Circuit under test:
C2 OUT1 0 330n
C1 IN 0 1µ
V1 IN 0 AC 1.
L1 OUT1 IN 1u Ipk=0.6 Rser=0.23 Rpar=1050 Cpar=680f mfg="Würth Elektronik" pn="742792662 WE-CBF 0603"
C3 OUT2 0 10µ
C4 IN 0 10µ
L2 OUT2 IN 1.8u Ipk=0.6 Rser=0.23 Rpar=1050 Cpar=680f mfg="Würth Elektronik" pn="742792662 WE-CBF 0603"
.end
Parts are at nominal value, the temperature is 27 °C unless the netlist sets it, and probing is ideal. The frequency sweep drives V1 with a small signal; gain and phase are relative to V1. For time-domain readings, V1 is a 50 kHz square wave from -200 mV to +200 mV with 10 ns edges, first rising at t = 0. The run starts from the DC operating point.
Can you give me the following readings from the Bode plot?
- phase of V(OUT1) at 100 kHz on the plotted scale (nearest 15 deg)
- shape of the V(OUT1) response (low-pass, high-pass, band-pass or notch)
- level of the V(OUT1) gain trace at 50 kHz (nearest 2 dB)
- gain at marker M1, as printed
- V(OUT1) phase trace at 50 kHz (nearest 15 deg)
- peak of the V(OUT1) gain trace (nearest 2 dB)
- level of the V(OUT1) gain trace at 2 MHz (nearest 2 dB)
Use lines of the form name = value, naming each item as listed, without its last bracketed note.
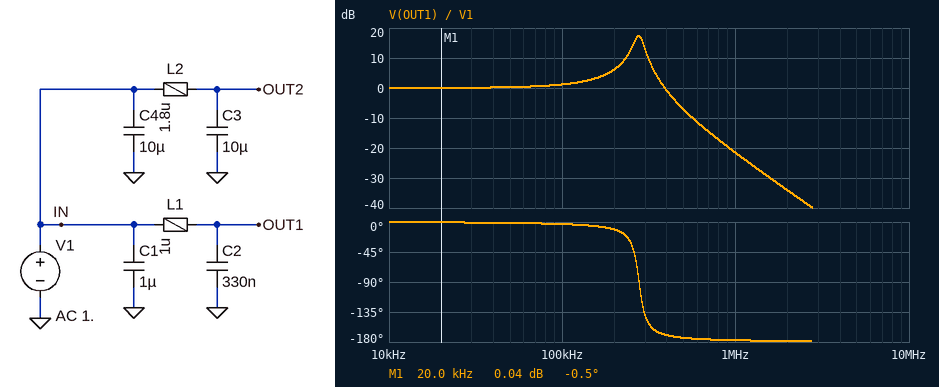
phase of V(OUT1) at 100 kHz on the plotted scale = 0 deg
shape of the V(OUT1) response = low-pass
level of the V(OUT1) gain trace at 50 kHz = 0 dB
gain at marker M1, as printed = 0.04 dB
V(OUT1) phase trace at 50 kHz = 0 deg
peak of the V(OUT1) gain trace = 18 dB
level of the V(OUT1) gain trace at 2 MHz = -34 dB
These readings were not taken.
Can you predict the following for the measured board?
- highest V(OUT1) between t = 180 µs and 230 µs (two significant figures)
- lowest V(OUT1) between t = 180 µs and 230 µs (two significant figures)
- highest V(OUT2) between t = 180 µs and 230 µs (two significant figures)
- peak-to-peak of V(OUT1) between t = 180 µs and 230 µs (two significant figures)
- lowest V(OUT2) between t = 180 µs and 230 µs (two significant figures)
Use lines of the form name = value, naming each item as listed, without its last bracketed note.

highest V(OUT1) between t = 180 µs and 230 µs = 510 mV
lowest V(OUT1) between t = 180 µs and 230 µs = -510 mV
highest V(OUT2) between t = 180 µs and 230 µs = 240 mV
peak-to-peak of V(OUT1) between t = 180 µs and 230 µs = 1.0 V
lowest V(OUT2) between t = 180 µs and 230 µs = -240 mV
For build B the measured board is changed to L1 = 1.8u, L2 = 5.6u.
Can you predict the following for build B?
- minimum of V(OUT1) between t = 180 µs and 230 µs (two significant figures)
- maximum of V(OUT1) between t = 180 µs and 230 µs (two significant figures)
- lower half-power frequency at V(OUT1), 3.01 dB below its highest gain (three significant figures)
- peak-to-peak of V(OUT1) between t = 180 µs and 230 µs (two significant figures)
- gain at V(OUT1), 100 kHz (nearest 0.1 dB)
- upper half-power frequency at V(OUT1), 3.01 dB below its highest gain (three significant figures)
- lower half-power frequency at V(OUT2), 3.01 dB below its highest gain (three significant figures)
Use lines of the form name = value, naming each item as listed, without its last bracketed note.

minimum of V(OUT1) between t = 180 µs and 230 µs = -430 mV
maximum of V(OUT1) between t = 180 µs and 230 µs = 430 mV
lower half-power frequency at V(OUT1), 3.01 dB below its highest gain = 195 kHz
peak-to-peak of V(OUT1) between t = 180 µs and 230 µs = 850 mV
gain at V(OUT1), 100 kHz = 2.3 dB
upper half-power frequency at V(OUT1), 3.01 dB below its highest gain = 216 kHz
lower half-power frequency at V(OUT2), 3.01 dB below its highest gain = 17.1 kHz
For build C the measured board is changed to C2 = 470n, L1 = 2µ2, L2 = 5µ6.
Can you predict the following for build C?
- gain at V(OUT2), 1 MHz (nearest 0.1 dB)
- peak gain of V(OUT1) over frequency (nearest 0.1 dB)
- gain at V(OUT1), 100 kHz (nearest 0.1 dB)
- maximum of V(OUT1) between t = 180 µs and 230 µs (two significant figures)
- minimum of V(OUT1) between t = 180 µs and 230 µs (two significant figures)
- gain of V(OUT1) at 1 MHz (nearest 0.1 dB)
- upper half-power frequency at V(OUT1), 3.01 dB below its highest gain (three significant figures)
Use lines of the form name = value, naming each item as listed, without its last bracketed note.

gain at V(OUT2), 1 MHz = -66.9 dB
peak gain of V(OUT1) over frequency = 19.3 dB
gain at V(OUT1), 100 kHz = 4.5 dB
maximum of V(OUT1) between t = 180 µs and 230 µs = 880 mV
minimum of V(OUT1) between t = 180 µs and 230 µs = -880 mV
gain of V(OUT1) at 1 MHz = -32.0 dB
upper half-power frequency at V(OUT1), 3.01 dB below its highest gain = 164 kHz
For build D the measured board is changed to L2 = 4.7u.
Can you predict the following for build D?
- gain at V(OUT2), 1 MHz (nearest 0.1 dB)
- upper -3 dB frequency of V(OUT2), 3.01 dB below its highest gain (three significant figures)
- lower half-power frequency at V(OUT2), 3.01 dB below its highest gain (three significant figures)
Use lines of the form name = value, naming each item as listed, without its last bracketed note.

gain at V(OUT2), 1 MHz = -65.4 dB
upper -3 dB frequency of V(OUT2), 3.01 dB below its highest gain = 26.2 kHz
lower half-power frequency at V(OUT2), 3.01 dB below its highest gain = 18.2 kHz
